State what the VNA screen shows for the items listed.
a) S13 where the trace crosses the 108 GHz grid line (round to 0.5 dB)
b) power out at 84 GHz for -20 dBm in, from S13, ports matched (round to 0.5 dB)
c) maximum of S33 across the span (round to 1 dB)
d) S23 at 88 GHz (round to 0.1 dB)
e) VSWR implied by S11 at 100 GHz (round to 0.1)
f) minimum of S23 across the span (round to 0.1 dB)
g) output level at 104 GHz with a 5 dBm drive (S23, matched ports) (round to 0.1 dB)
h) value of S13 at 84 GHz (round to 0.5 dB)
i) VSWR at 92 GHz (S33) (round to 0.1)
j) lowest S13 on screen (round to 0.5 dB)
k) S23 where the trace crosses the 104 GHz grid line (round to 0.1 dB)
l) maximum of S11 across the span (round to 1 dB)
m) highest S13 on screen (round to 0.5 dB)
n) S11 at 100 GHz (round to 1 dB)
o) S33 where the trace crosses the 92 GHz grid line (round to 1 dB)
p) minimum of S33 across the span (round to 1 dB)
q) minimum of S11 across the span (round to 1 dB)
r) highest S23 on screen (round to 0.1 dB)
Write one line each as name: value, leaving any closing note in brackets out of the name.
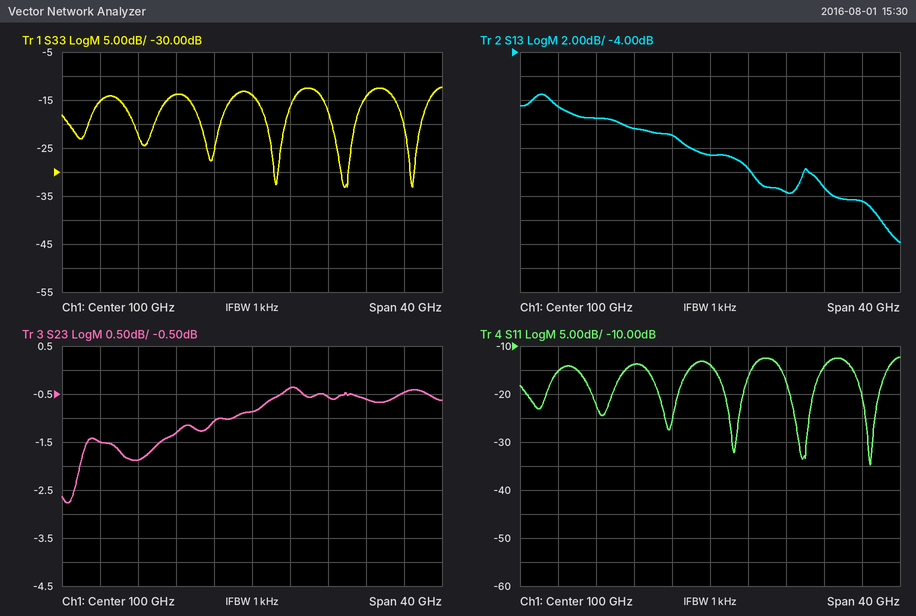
S13 where the trace crosses the 108 GHz grid line: -15.5 dB
power out at 84 GHz for -20 dBm in, from S13, ports matched: -28.5 dBm
maximum of S33 across the span: -12 dB
S23 at 88 GHz: -1.9 dB
VSWR implied by S11 at 100 GHz: 1.5
minimum of S23 across the span: -2.8 dB
output level at 104 GHz with a 5 dBm drive (S23, matched ports): 4.6 dBm
value of S13 at 84 GHz: -8.5 dB
VSWR at 92 GHz (S33): 1.5
lowest S13 on screen: -20.0 dB
S23 where the trace crosses the 104 GHz grid line: -0.4 dB
maximum of S11 across the span: -12 dB
highest S13 on screen: -7.5 dB
S11 at 100 GHz: -14 dB
S33 where the trace crosses the 92 GHz grid line: -14 dB
minimum of S33 across the span: -33 dB
minimum of S11 across the span: -35 dB
highest S23 on screen: -0.4 dB
